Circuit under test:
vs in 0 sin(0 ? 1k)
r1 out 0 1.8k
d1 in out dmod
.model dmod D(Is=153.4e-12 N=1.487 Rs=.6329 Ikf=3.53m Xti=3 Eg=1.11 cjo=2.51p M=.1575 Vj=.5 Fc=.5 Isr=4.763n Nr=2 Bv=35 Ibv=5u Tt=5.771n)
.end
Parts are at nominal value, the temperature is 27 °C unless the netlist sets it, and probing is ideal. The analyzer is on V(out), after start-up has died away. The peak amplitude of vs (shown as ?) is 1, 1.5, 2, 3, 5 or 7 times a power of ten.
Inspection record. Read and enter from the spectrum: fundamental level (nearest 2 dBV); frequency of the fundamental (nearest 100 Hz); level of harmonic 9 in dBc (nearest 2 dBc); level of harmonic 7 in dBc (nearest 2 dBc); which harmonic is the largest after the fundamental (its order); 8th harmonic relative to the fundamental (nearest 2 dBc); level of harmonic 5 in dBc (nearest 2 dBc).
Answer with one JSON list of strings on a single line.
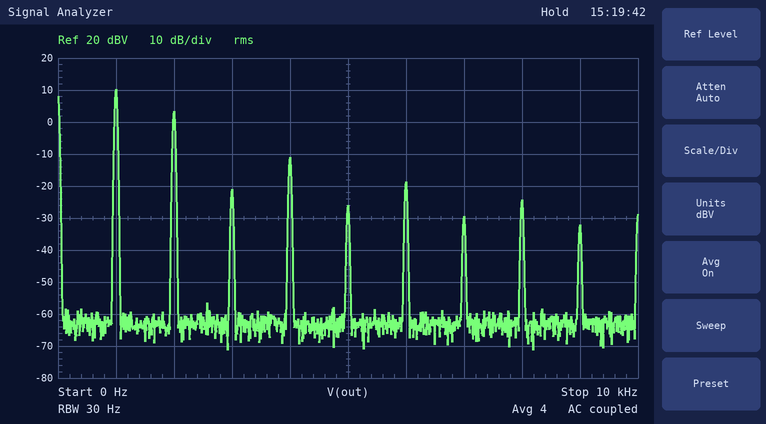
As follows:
["10 dBV", "1.0 kHz", "-42 dBc", "-40 dBc", "2", "-34 dBc", "-36 dBc"]
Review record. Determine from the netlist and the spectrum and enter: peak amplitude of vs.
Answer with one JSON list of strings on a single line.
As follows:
["10 V"]
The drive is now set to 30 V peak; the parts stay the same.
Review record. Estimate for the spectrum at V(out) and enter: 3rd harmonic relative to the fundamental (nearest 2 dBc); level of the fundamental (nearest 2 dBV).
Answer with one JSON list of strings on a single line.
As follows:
["-40 dBc", "20 dBV"]
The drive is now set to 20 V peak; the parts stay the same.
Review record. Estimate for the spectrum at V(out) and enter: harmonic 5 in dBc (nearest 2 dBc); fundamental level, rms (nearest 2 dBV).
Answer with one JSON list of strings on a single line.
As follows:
["-42 dBc", "16 dBV"]
